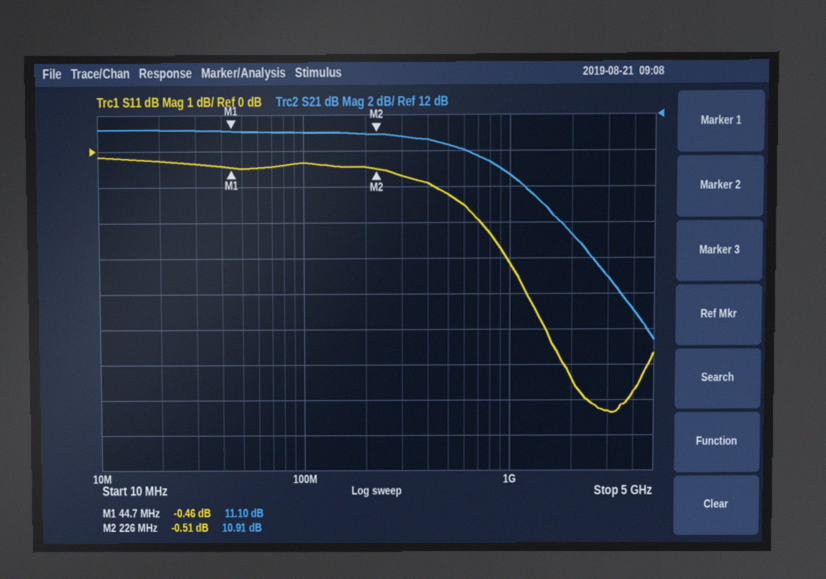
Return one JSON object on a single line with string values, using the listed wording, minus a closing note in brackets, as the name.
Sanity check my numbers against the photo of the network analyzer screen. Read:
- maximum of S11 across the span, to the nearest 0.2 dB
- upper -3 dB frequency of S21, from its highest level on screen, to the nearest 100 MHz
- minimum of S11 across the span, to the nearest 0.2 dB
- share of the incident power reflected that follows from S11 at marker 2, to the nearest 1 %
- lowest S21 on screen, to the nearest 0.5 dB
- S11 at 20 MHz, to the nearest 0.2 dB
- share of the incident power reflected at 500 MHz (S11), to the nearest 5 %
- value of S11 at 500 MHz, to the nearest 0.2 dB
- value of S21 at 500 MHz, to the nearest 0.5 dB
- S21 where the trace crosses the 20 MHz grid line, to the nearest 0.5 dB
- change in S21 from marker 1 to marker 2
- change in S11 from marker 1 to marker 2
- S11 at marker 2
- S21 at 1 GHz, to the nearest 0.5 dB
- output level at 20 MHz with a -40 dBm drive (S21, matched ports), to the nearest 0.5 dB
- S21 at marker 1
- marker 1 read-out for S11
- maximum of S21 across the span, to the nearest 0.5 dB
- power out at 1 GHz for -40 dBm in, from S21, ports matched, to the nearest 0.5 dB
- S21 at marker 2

{"maximum of S11 across the span, to the nearest 0.2 dB": "-0.2 dB", "upper -3 dB frequency of S21, from its highest level on screen, to the nearest 100 MHz": "1.1 GHz", "minimum of S11 across the span, to the nearest 0.2 dB": "-7.4 dB", "share of the incident power reflected that follows from S11 at marker 2, to the nearest 1 %": "89 %", "lowest S21 on screen, to the nearest 0.5 dB": "-0.5 dB", "S11 at 20 MHz, to the nearest 0.2 dB": "-0.2 dB", "share of the incident power reflected at 500 MHz (S11), to the nearest 5 %": "75 %", "value of S11 at 500 MHz, to the nearest 0.2 dB": "-1.2 dB", "value of S21 at 500 MHz, to the nearest 0.5 dB": "10.5 dB", "S21 where the trace crosses the 20 MHz grid line, to the nearest 0.5 dB": "11.0 dB", "change in S21 from marker 1 to marker 2": "-0.19 dB", "change in S11 from marker 1 to marker 2": "-0.05 dB", "S11 at marker 2": "-0.51 dB", "S21 at 1 GHz, to the nearest 0.5 dB": "8.5 dB", "output level at 20 MHz with a -40 dBm drive (S21, matched ports), to the nearest 0.5 dB": "-29.0 dBm", "S21 at marker 1": "11.10 dB", "marker 1 read-out for S11": "-0.46 dB", "maximum of S21 across the span, to the nearest 0.5 dB": "11.0 dB", "power out at 1 GHz for -40 dBm in, from S21, ports matched, to the nearest 0.5 dB": "-31.5 dBm", "S21 at marker 2": "10.91 dB"}
